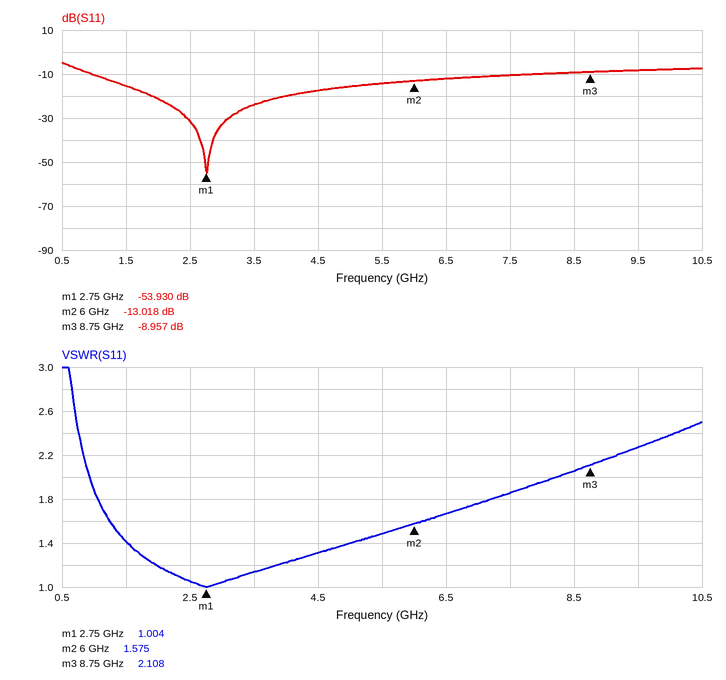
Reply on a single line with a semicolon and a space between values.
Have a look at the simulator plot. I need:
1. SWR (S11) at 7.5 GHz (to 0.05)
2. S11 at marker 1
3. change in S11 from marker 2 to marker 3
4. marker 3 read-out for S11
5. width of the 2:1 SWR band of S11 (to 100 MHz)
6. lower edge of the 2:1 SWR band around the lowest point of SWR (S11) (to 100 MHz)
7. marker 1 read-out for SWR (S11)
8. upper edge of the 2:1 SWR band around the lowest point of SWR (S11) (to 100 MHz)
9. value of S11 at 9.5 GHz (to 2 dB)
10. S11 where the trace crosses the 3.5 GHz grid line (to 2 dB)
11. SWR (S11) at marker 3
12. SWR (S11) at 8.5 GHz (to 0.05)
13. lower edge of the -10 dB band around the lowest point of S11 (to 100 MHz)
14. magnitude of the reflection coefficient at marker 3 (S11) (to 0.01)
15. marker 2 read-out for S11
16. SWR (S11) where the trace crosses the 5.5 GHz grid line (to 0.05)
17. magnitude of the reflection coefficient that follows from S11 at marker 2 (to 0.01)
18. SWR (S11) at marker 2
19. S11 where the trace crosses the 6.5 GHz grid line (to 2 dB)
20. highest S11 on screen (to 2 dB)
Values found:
1.85; -53.930 dB; 4.061 dB; -8.957 dB; 7.3 GHz; 900 MHz; 1.004; 8.2 GHz; -8 dB; -24 dB; 2.108; 2.05; 1.0 GHz; 0.36; -13.018 dB; 1.50; 0.22; 1.575; -12 dB; -4 dB
